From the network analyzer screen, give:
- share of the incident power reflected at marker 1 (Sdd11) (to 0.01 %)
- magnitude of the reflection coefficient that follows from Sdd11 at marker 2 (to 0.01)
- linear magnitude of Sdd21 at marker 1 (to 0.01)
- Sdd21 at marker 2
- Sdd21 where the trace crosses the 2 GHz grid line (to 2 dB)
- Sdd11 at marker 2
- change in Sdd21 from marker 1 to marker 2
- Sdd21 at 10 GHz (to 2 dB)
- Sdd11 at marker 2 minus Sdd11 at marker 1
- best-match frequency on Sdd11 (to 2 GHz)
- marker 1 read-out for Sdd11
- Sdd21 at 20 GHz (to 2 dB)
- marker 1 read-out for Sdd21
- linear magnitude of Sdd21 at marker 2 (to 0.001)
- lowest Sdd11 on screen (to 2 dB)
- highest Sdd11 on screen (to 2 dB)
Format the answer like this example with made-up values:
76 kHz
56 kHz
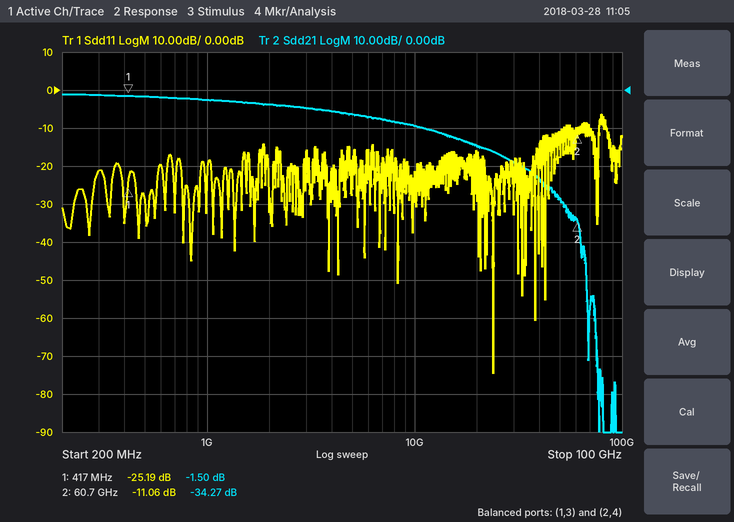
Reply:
0.30 %
0.28
0.84
-34.27 dB
-4 dB
-11.06 dB
-32.77 dB
-10 dB
14.13 dB
24 GHz
-25.19 dB
-14 dB
-1.50 dB
0.019
-74 dB
-6 dB
